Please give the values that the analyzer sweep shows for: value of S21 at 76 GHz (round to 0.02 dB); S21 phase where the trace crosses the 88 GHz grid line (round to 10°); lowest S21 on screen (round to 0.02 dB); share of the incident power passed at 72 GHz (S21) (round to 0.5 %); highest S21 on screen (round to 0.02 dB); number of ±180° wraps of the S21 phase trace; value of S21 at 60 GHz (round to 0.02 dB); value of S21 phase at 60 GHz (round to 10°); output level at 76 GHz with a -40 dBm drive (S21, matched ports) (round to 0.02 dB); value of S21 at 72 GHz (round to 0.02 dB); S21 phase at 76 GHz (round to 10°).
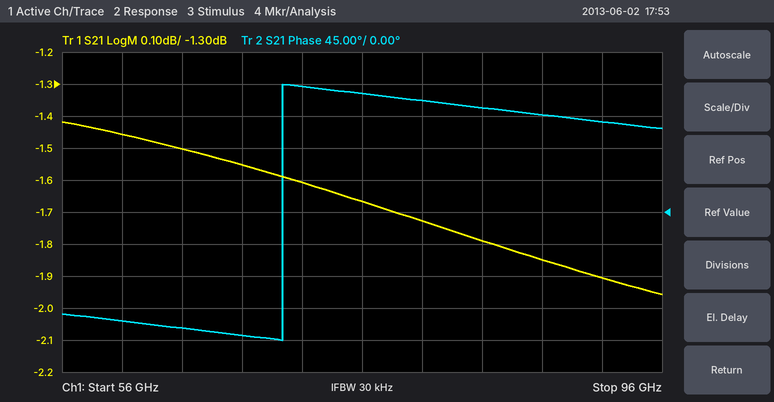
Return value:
-1.66 dB
140°
-1.96 dB
69.0 %
-1.42 dB
1
-1.46 dB
-150°
-41.66 dBm
-1.60 dB
170°
